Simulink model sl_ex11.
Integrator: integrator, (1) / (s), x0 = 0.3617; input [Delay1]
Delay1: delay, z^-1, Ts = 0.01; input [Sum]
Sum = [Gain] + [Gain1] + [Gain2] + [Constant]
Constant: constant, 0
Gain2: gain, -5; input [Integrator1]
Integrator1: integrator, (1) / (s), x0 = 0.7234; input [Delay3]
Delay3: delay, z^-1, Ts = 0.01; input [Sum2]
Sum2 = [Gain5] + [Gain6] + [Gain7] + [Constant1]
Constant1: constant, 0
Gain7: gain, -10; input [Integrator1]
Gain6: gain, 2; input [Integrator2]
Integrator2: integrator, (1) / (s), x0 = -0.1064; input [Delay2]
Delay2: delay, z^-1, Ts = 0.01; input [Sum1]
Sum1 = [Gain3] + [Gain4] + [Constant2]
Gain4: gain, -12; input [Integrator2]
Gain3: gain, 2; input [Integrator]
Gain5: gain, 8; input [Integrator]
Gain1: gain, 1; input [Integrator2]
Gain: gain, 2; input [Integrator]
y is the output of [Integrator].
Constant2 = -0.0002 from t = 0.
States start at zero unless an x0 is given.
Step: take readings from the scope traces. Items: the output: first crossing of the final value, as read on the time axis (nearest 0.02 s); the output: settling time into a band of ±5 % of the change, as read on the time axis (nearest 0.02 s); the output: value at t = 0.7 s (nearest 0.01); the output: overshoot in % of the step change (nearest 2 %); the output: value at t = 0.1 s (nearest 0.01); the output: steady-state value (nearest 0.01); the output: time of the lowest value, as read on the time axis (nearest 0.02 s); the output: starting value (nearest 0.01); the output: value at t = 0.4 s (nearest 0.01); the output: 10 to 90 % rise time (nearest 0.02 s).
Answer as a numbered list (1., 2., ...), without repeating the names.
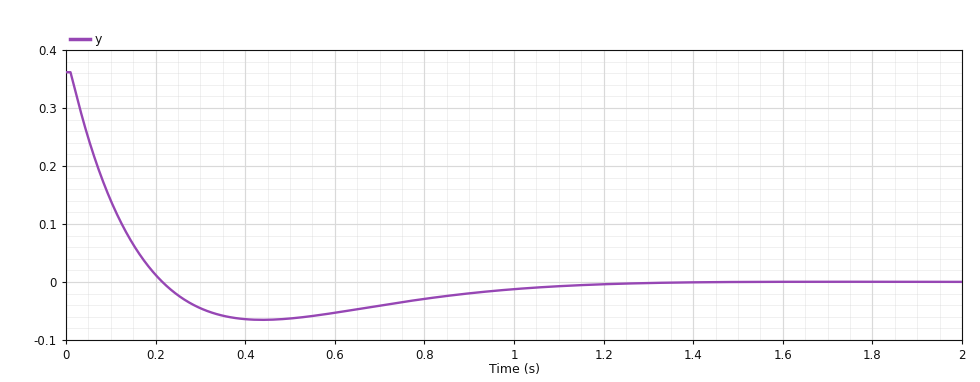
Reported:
1. 0.22 s
2. 0.92 s
3. -0.04
4. 18 %
5. 0.14
6. 0.00
7. 0.44 s
8. 0.36
9. -0.06
10. 0.16 s
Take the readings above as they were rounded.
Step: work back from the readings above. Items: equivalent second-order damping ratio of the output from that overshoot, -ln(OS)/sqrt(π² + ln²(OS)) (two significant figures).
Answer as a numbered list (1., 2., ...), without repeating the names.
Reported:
1. 0.48
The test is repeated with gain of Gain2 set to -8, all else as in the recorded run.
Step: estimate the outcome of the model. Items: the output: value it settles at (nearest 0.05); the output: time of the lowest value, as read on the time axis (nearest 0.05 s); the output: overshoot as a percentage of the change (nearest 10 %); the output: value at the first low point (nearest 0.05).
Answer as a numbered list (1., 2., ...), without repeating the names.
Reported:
1. 0.00
2. 0.25 s
3. 70 %
4. -0.25
